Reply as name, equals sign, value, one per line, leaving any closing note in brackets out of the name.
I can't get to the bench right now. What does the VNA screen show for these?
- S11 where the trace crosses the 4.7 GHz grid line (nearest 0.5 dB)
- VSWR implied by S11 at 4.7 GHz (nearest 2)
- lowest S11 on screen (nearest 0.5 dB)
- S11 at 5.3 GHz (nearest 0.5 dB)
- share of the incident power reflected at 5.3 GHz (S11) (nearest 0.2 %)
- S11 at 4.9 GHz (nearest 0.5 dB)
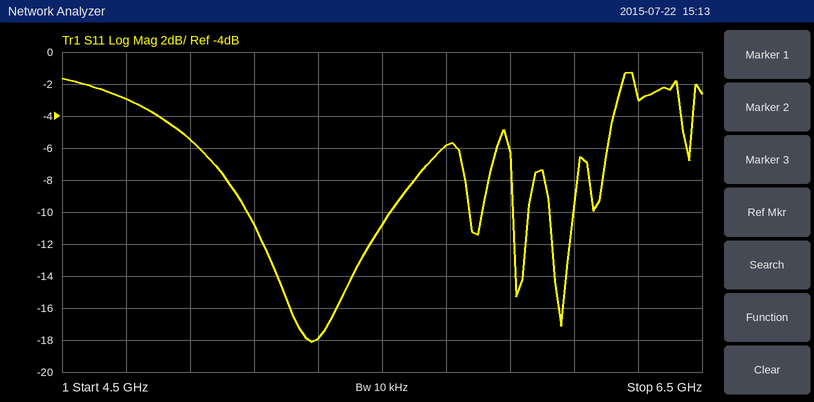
S11 where the trace crosses the 4.7 GHz grid line = -3.0 dB
VSWR implied by S11 at 4.7 GHz = 6
lowest S11 on screen = -18.0 dB
S11 at 5.3 GHz = -18.0 dB
share of the incident power reflected at 5.3 GHz (S11) = 1.6 %
S11 at 4.9 GHz = -5.5 dB
